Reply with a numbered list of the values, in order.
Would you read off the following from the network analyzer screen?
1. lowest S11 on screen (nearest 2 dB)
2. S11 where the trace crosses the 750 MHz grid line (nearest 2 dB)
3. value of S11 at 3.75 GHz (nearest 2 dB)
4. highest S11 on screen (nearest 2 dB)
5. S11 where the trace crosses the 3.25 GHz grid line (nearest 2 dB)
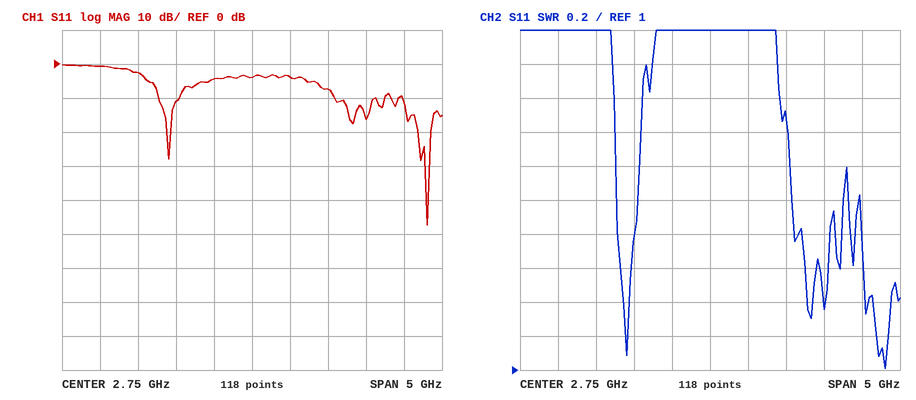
1. -48 dB
2. 0 dB
3. -8 dB
4. 0 dB
5. -4 dB
